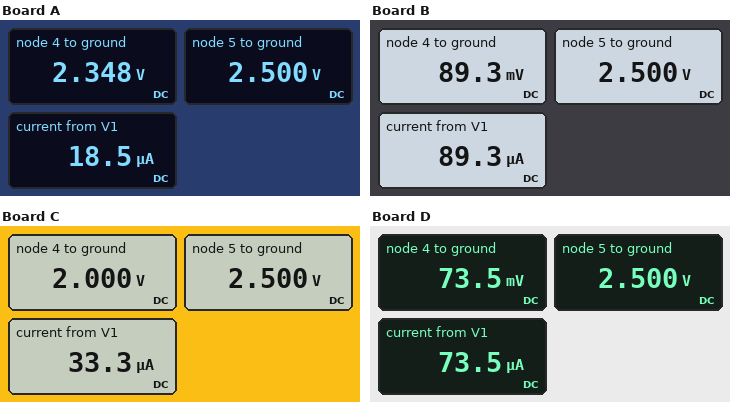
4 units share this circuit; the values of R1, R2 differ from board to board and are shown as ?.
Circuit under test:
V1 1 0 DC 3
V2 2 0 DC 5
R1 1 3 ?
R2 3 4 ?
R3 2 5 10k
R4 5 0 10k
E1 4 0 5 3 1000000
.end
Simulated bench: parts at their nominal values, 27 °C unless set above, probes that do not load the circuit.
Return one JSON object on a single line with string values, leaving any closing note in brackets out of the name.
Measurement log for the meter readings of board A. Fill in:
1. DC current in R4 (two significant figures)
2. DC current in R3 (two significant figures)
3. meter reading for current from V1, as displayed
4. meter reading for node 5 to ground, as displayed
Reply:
{"DC current in R4": "250 µA", "DC current in R3": "250 µA", "meter reading for current from V1, as displayed": "18.5 µA", "meter reading for node 5 to ground, as displayed": "2.500 V"}
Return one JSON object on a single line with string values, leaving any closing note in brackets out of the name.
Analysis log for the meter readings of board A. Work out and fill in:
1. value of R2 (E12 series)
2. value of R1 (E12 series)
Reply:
{"value of R2": "8.2 kΩ", "value of R1": "27 kΩ"}
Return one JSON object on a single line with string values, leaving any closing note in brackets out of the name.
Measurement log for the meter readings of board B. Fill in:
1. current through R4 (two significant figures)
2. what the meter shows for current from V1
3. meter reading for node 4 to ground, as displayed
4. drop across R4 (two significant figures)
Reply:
{"current through R4": "250 µA", "what the meter shows for current from V1": "89.3 µA", "meter reading for node 4 to ground, as displayed": "89.3 mV", "drop across R4": "2.5 V"}
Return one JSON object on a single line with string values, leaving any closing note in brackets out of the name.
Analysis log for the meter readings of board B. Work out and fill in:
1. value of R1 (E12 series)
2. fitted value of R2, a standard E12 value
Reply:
{"value of R1": "5.6 kΩ", "fitted value of R2, a standard E12 value": "27 kΩ"}
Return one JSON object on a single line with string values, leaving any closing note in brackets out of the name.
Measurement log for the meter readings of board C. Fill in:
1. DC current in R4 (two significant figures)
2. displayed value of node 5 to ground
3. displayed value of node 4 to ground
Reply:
{"DC current in R4": "250 µA", "displayed value of node 5 to ground": "2.500 V", "displayed value of node 4 to ground": "2.000 V"}
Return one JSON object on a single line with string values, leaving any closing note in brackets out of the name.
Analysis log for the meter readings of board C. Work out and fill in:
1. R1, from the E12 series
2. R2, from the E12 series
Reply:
{"R1, from the E12 series": "15 kΩ", "R2, from the E12 series": "15 kΩ"}
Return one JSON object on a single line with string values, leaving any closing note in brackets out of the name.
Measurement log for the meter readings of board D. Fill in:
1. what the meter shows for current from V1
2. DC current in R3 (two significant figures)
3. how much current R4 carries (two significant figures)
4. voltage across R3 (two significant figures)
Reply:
{"what the meter shows for current from V1": "73.5 µA", "DC current in R3": "250 µA", "how much current R4 carries": "250 µA", "voltage across R3": "2.5 V"}
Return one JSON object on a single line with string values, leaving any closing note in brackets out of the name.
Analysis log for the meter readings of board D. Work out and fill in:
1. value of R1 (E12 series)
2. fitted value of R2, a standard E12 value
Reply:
{"value of R1": "6.8 kΩ", "fitted value of R2, a standard E12 value": "33 kΩ"}
